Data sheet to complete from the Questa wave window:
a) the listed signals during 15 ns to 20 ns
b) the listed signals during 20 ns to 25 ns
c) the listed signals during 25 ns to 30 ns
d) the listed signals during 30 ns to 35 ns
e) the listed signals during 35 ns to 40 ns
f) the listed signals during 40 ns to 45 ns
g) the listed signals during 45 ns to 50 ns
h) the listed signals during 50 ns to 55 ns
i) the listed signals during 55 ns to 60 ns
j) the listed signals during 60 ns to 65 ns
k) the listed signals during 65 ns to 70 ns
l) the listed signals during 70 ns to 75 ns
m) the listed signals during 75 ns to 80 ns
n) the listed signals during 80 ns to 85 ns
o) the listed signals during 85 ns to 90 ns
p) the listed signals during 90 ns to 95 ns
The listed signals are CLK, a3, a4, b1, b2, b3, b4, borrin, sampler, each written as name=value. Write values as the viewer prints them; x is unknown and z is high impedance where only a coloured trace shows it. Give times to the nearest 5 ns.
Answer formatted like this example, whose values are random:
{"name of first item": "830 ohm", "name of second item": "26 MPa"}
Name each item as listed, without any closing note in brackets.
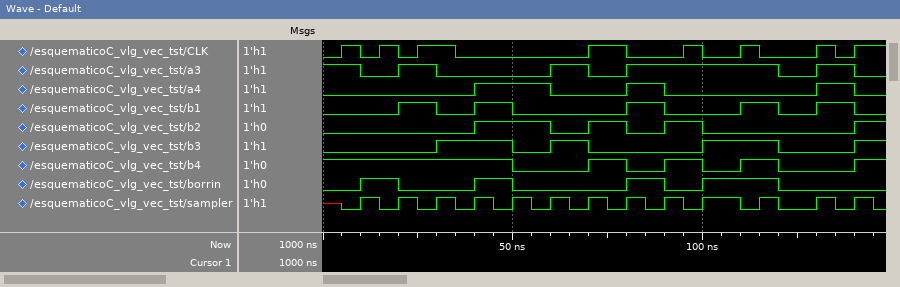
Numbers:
{"the listed signals during 15 ns to 20 ns": "CLK=1, a3=0, a4=0, b1=0, b2=0, b3=0, b4=1, borrin=1, sampler=0", "the listed signals during 20 ns to 25 ns": "CLK=0, a3=1, a4=0, b1=1, b2=0, b3=0, b4=1, borrin=0, sampler=1", "the listed signals during 25 ns to 30 ns": "CLK=1, a3=1, a4=0, b1=1, b2=0, b3=0, b4=1, borrin=0, sampler=0", "the listed signals during 30 ns to 35 ns": "CLK=1, a3=0, a4=0, b1=0, b2=0, b3=1, b4=1, borrin=0, sampler=1", "the listed signals during 35 ns to 40 ns": "CLK=0, a3=0, a4=0, b1=0, b2=0, b3=1, b4=1, borrin=0, sampler=0", "the listed signals during 40 ns to 45 ns": "CLK=0, a3=0, a4=1, b1=1, b2=1, b3=1, b4=1, borrin=1, sampler=1", "the listed signals during 45 ns to 50 ns": "CLK=0, a3=0, a4=1, b1=1, b2=1, b3=1, b4=1, borrin=1, sampler=0", "the listed signals during 50 ns to 55 ns": "CLK=0, a3=0, a4=1, b1=0, b2=1, b3=0, b4=0, borrin=0, sampler=1", "the listed signals during 55 ns to 60 ns": "CLK=0, a3=0, a4=1, b1=0, b2=1, b3=0, b4=0, borrin=0, sampler=0", "the listed signals during 60 ns to 65 ns": "CLK=0, a3=1, a4=0, b1=0, b2=0, b3=1, b4=0, borrin=0, sampler=1", "the listed signals during 65 ns to 70 ns": "CLK=0, a3=1, a4=0, b1=0, b2=0, b3=1, b4=0, borrin=0, sampler=0", "the listed signals during 70 ns to 75 ns": "CLK=1, a3=0, a4=0, b1=0, b2=1, b3=0, b4=1, borrin=0, sampler=1", "the listed signals during 75 ns to 80 ns": "CLK=1, a3=0, a4=0, b1=0, b2=1, b3=0, b4=1, borrin=0, sampler=0", "the listed signals during 80 ns to 85 ns": "CLK=0, a3=1, a4=1, b1=1, b2=0, b3=0, b4=0, borrin=1, sampler=1", "the listed signals during 85 ns to 90 ns": "CLK=0, a3=1, a4=1, b1=1, b2=0, b3=0, b4=0, borrin=1, sampler=0", "the listed signals during 90 ns to 95 ns": "CLK=0, a3=1, a4=0, b1=0, b2=1, b3=0, b4=1, borrin=0, sampler=1"}
